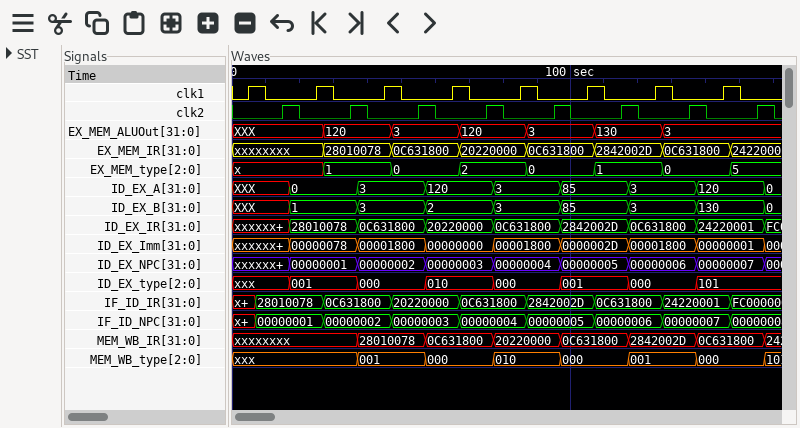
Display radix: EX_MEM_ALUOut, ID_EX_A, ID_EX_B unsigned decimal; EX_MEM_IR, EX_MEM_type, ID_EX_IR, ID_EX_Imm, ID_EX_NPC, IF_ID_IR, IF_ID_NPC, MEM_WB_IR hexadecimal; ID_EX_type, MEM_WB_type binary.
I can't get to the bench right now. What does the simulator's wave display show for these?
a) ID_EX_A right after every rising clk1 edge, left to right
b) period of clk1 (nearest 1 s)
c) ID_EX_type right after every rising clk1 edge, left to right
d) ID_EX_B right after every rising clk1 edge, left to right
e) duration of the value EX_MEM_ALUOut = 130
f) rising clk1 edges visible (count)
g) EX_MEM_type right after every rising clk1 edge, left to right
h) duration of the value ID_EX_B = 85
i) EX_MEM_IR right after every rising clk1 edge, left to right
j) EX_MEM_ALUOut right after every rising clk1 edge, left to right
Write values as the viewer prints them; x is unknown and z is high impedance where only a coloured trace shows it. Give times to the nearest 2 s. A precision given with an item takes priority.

XXX, 0, 3, 120, 3, 85, 3, 120
20 s
xxx, 001, 000, 010, 000, 001, 000, 101
XXX, 1, 3, 2, 3, 85, 3, 130
20 s
8
x, x, 1, 0, 2, 0, 1, 0
20 s
xxxxxxxx, xxxxxxxx, 28010078, 0C631800, 20220000, 0C631800, 2842002D, 0C631800
XXX, XXX, 120, 3, 120, 3, 130, 3
